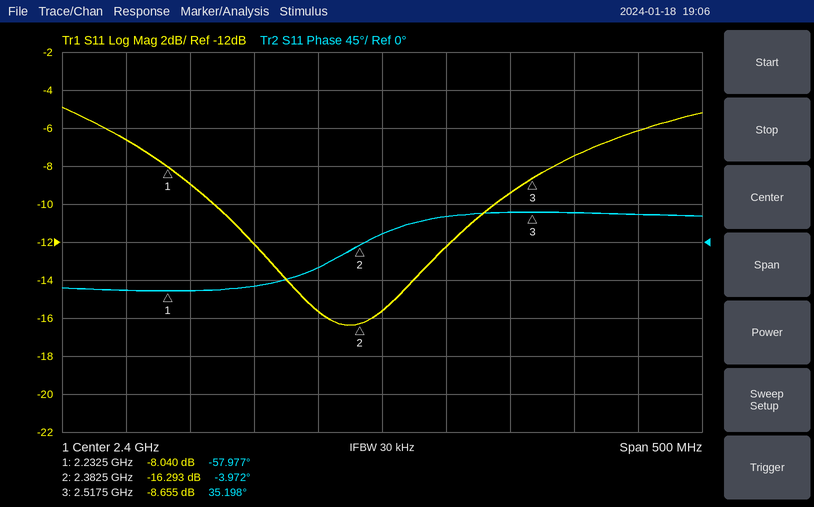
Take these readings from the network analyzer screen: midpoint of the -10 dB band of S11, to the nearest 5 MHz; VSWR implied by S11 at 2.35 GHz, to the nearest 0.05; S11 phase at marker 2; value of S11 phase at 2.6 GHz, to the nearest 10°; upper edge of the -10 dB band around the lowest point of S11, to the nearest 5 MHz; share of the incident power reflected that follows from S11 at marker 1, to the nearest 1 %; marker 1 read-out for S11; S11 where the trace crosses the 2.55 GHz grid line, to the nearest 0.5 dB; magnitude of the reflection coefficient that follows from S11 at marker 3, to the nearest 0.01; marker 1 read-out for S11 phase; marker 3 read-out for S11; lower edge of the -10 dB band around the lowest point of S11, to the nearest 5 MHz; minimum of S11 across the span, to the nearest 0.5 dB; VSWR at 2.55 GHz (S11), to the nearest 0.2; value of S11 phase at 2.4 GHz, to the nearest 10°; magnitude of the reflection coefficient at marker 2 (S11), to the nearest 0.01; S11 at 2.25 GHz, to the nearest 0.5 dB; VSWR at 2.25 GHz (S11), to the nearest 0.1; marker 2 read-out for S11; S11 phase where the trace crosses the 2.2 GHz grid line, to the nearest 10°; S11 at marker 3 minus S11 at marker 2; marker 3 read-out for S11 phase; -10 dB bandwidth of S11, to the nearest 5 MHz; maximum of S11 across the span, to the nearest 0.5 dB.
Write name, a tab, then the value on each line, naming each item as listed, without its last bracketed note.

midpoint of the -10 dB band of S11, to the nearest 5 MHz	2.380 GHz
VSWR implied by S11 at 2.35 GHz, to the nearest 0.05	1.40
S11 phase at marker 2	-3.972°
value of S11 phase at 2.6 GHz, to the nearest 10°	30°
upper edge of the -10 dB band around the lowest point of S11, to the nearest 5 MHz	2.490 GHz
share of the incident power reflected that follows from S11 at marker 1, to the nearest 1 %	16 %
marker 1 read-out for S11	-8.040 dB
S11 where the trace crosses the 2.55 GHz grid line, to the nearest 0.5 dB	-7.5 dB
magnitude of the reflection coefficient that follows from S11 at marker 3, to the nearest 0.01	0.37
marker 1 read-out for S11 phase	-57.977°
marker 3 read-out for S11	-8.655 dB
lower edge of the -10 dB band around the lowest point of S11, to the nearest 5 MHz	2.270 GHz
minimum of S11 across the span, to the nearest 0.5 dB	-16.5 dB
VSWR at 2.55 GHz (S11), to the nearest 0.2	2.4
value of S11 phase at 2.4 GHz, to the nearest 10°	10°
magnitude of the reflection coefficient at marker 2 (S11), to the nearest 0.01	0.15
S11 at 2.25 GHz, to the nearest 0.5 dB	-9.0 dB
VSWR at 2.25 GHz (S11), to the nearest 0.1	2.1
marker 2 read-out for S11	-16.293 dB
S11 phase where the trace crosses the 2.2 GHz grid line, to the nearest 10°	-60°
S11 at marker 3 minus S11 at marker 2	7.638 dB
marker 3 read-out for S11 phase	35.198°
-10 dB bandwidth of S11, to the nearest 5 MHz	220 MHz
maximum of S11 across the span, to the nearest 0.5 dB	-5.0 dB
